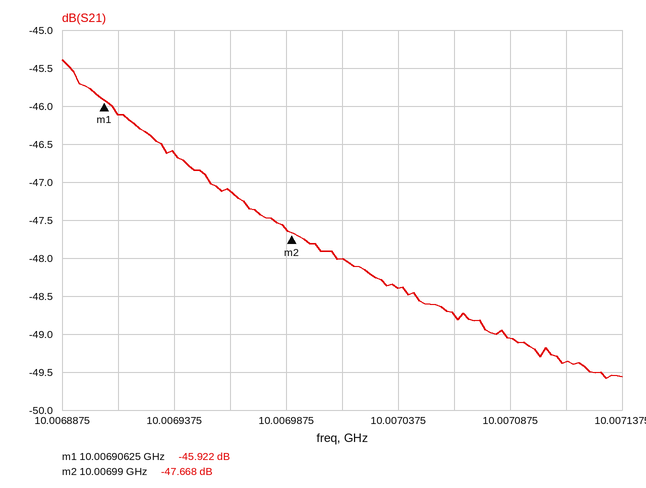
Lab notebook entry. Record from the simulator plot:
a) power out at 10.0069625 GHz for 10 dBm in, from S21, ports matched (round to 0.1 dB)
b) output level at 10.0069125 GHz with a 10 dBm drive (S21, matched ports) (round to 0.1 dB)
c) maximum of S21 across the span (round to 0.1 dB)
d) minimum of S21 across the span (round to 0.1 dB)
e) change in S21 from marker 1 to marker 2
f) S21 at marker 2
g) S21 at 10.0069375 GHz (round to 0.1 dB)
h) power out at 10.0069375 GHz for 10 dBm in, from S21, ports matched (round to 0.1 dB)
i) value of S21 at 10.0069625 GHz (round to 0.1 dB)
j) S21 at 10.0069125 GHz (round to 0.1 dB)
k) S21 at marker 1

-37.1 dBm
-36.1 dBm
-45.4 dB
-49.6 dB
-1.746 dB
-47.668 dB
-46.6 dB
-36.6 dBm
-47.1 dB
-46.1 dB
-45.922 dB
